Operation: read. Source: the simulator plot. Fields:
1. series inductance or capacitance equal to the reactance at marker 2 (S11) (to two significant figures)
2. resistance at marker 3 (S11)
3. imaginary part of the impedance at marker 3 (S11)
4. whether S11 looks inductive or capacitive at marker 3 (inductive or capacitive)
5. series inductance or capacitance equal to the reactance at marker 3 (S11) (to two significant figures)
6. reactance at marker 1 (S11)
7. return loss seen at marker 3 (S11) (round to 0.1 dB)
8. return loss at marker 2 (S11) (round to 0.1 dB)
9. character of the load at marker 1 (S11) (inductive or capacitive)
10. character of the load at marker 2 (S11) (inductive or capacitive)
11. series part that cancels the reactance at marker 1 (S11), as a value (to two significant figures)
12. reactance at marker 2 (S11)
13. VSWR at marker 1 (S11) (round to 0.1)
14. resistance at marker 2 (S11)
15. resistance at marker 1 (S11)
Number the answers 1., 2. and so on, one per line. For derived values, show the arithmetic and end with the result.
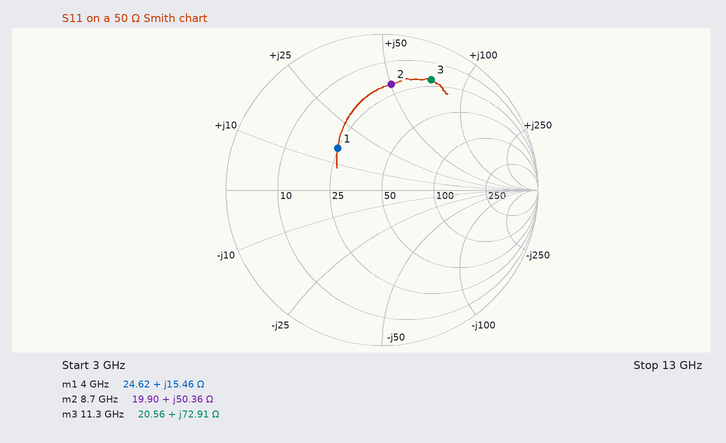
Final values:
1. L = 50.36 Ω/(2π × 8.7 GHz) ≈ 921 pH, so 920 pH to two significant figures
2. 20.56 Ω
3. +72.91 Ω
4. inductive
5. L = 72.91 Ω/(2π × 11.3 GHz) ≈ 1.0 nH
6. +15.46 Ω
7. 2.2 dB
8. 3.3 dB
9. inductive
10. inductive
11. C = 1/(2π × 4 GHz × 15.46 Ω) ≈ 2.6 pF
12. +50.36 Ω
13. 2.3
14. 19.90 Ω
15. 24.62 Ω
